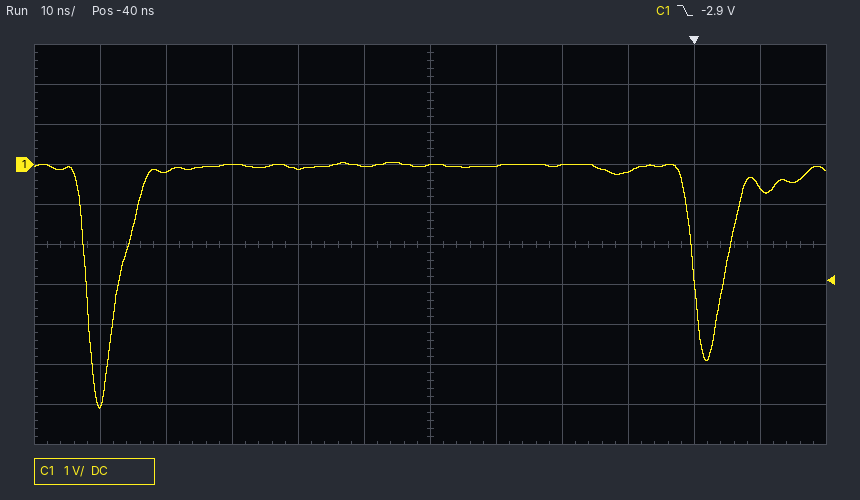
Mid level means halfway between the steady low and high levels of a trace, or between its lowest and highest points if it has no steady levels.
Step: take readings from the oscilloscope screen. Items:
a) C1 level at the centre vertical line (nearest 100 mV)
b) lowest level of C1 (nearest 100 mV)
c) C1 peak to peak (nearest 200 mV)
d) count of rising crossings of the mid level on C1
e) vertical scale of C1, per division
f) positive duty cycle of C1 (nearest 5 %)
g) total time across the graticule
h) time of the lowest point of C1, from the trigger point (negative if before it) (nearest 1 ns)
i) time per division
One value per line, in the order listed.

0.0 V
-6.1 V
6.2 V
2
1 V
95 %
120 ns
-90 ns
10 ns
